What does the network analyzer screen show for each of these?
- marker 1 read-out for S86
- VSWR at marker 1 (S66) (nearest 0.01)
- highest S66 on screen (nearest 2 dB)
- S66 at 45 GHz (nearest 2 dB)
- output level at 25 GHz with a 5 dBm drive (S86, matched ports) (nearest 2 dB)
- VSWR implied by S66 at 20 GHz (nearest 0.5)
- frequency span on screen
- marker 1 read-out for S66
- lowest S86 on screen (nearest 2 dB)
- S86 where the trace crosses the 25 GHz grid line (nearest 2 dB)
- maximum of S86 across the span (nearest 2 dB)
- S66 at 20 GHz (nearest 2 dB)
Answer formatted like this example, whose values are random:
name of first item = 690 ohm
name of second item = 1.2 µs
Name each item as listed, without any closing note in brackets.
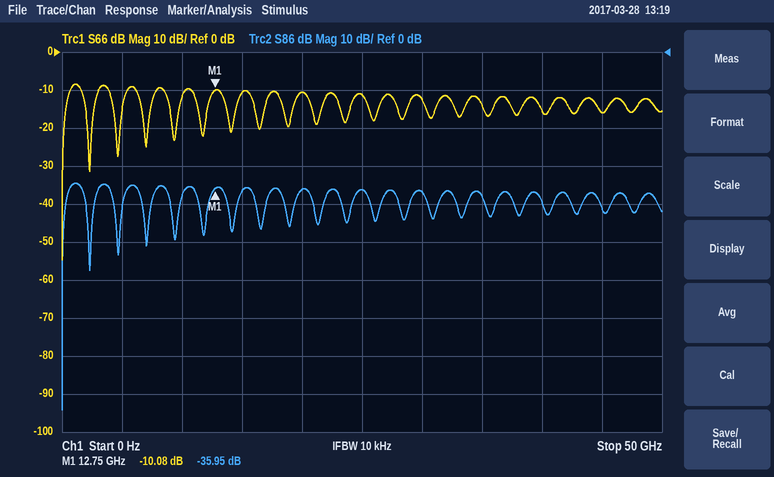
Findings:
marker 1 read-out for S86 = -35.95 dB
VSWR at marker 1 (S66) = 1.91
highest S66 on screen = -8 dB
S66 at 45 GHz = -16 dB
output level at 25 GHz with a 5 dBm drive (S86, matched ports) = -32 dBm
VSWR implied by S66 at 20 GHz = 2.0
frequency span on screen = 50 GHz
marker 1 read-out for S66 = -10.08 dB
lowest S86 on screen = -94 dB
S86 where the trace crosses the 25 GHz grid line = -36 dB
maximum of S86 across the span = -34 dB
S66 at 20 GHz = -10 dB
